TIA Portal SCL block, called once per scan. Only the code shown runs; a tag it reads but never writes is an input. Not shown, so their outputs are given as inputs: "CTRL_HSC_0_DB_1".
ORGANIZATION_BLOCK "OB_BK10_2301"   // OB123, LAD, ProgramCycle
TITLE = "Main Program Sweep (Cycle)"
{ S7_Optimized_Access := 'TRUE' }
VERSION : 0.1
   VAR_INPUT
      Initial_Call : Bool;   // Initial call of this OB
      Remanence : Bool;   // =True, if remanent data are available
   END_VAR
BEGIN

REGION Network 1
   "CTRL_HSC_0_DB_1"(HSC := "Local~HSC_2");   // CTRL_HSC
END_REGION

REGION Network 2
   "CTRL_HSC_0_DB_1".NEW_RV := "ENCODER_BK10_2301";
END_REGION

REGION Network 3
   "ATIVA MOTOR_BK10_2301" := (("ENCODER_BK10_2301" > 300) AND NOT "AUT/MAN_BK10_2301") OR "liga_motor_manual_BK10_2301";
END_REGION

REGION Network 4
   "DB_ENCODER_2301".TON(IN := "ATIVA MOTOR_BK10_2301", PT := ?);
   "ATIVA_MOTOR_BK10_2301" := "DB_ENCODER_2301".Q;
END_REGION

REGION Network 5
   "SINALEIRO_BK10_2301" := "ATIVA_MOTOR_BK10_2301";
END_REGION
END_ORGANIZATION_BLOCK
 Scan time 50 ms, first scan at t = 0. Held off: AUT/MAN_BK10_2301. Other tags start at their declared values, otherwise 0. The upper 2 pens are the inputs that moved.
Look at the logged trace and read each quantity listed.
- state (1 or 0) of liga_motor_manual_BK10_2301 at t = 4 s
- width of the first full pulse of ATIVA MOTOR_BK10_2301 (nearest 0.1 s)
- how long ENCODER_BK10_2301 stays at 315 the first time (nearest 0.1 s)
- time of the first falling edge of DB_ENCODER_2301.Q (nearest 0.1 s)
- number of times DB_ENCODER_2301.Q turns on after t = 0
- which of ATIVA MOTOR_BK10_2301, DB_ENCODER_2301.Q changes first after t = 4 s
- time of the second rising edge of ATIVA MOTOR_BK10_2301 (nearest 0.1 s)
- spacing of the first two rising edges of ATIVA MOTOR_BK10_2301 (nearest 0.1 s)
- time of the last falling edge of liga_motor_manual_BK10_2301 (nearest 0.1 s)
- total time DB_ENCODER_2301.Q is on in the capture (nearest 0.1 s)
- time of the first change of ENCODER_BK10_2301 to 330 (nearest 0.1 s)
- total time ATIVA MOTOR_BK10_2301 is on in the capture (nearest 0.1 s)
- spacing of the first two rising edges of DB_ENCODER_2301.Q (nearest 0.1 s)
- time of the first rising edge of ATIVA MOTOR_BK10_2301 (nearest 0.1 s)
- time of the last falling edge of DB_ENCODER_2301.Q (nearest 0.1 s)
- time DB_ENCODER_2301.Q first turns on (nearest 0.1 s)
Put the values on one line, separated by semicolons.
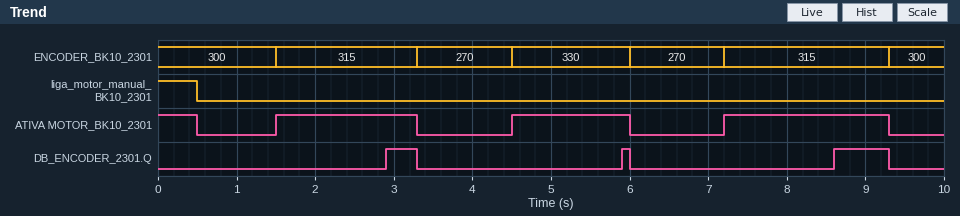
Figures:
0; 1.8 s; 1.8 s; 3.3 s; 3; ATIVA MOTOR_BK10_2301; 4.5 s; 3.0 s; 0.5 s; 1.2 s; 4.5 s; 5.9 s; 3.0 s; 1.5 s; 9.3 s; 2.9 s
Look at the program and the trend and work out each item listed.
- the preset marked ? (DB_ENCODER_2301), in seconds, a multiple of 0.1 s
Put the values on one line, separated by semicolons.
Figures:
1.4 s
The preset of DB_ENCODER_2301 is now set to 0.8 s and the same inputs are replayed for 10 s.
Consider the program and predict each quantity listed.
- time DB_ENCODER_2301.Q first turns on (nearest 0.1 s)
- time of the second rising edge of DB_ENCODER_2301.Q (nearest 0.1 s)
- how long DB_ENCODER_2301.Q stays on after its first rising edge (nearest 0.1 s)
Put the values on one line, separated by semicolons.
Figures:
2.3 s; 5.3 s; 1.0 s
